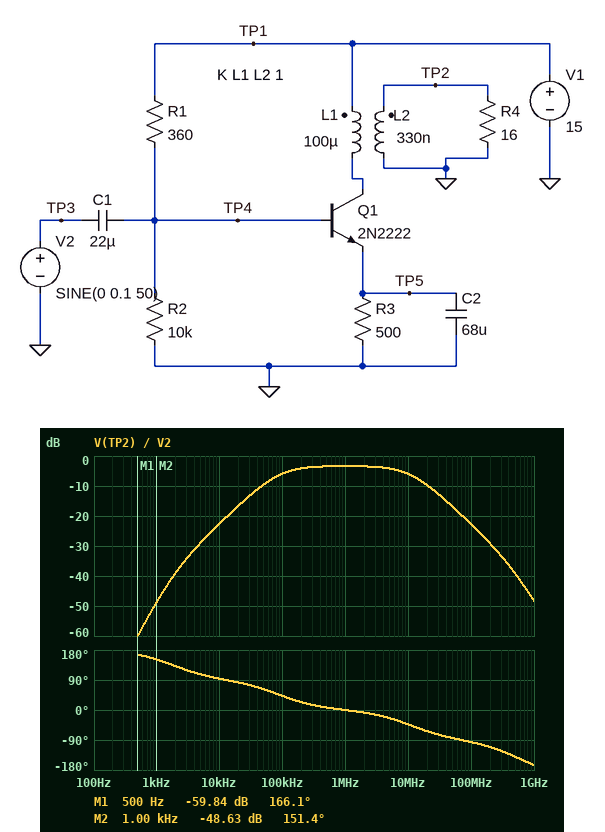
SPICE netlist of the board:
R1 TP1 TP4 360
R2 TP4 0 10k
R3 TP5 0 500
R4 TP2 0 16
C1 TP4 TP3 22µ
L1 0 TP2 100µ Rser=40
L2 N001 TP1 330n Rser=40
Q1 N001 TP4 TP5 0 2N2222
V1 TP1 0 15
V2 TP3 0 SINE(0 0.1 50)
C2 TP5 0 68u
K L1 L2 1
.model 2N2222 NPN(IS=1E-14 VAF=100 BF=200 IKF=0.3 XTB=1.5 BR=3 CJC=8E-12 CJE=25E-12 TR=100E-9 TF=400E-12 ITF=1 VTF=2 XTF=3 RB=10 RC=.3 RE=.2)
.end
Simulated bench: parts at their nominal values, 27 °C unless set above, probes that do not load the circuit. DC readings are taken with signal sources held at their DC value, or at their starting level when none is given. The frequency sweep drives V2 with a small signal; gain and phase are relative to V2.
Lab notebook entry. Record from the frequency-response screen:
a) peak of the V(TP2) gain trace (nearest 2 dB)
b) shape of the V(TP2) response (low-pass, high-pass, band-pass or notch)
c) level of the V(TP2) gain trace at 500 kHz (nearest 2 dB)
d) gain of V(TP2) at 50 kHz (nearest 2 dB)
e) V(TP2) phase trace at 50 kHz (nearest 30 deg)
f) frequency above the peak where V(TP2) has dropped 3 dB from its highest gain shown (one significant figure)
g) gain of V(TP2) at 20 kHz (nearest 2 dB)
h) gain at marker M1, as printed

-4 dB
band-pass
-4 dB
-10 dB
60 deg
10 MHz
-16 dB
-59.84 dB
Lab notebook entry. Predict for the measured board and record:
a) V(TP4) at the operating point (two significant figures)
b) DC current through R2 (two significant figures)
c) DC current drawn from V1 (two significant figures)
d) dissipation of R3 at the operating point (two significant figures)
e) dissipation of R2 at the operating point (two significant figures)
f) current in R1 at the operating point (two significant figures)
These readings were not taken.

14 V
1.4 mA
29 mA
370 mW
21 mW
1.6 mA
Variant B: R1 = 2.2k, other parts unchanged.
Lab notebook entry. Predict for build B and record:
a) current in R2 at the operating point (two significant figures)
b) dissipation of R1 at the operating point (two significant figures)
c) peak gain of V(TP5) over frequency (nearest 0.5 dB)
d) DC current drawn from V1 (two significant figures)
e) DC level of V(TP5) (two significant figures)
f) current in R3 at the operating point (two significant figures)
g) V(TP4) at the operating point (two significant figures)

1.2 mA
3.9 mW
0 dB
24 mA
11 V
23 mA
12 V
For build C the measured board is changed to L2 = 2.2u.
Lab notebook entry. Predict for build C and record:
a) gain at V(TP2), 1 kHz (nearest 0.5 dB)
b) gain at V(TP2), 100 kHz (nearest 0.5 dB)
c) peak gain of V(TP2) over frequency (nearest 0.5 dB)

-40.5 dB
2.5 dB
5.0 dB
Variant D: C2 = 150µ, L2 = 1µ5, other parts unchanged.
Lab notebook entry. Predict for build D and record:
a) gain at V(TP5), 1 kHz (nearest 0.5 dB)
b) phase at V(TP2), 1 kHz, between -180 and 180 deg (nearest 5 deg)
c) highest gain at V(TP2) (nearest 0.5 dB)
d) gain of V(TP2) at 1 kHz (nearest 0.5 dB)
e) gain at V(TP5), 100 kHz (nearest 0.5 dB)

-4.5 dB
130 deg
3.0 dB
-38.0 dB
-42.0 dB
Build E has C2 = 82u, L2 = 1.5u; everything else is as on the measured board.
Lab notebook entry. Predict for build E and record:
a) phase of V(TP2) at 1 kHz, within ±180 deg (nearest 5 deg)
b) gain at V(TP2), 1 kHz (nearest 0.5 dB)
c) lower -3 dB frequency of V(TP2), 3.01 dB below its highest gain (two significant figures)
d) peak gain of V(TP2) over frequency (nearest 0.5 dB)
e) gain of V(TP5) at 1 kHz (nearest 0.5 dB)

145 deg
-41.0 dB
88 kHz
3.0 dB
-2.0 dB
